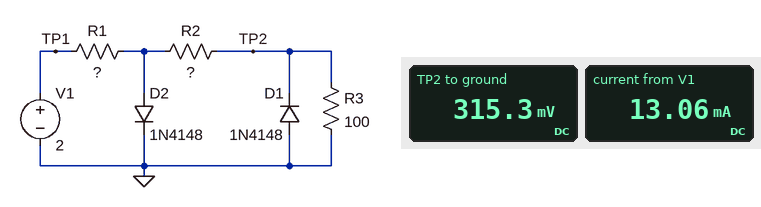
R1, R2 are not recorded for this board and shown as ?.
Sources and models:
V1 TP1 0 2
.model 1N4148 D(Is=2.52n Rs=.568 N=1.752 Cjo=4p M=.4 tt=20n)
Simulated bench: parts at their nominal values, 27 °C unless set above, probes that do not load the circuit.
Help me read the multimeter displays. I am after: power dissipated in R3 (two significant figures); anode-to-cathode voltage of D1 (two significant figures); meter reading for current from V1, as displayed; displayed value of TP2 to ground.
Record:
990 µW
-320 mV
13.06 mA
315.3 mV
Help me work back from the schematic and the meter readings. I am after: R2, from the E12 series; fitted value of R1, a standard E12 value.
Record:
120 Ω
100 Ω
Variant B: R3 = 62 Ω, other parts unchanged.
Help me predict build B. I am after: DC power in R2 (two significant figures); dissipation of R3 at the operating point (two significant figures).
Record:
1.7 mW
890 µW
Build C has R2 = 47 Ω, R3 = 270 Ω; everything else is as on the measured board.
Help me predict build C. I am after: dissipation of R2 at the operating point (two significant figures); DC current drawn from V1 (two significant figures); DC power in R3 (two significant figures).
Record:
230 µW
13 mA
1.3 mW
